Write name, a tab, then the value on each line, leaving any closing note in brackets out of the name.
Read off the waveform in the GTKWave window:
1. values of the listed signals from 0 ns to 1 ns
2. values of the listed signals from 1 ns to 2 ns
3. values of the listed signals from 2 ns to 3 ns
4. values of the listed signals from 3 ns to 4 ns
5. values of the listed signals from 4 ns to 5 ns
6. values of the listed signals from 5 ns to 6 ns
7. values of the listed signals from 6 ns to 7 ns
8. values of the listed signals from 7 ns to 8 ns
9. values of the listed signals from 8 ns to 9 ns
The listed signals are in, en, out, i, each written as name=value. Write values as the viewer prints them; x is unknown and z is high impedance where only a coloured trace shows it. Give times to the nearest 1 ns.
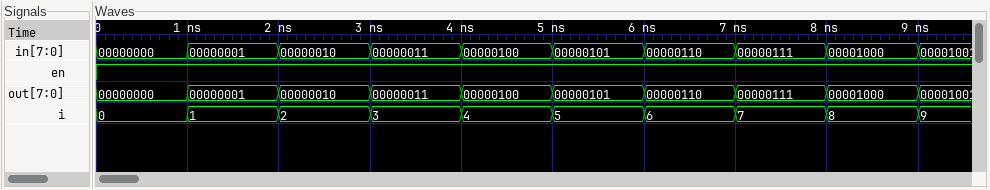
values of the listed signals from 0 ns to 1 ns	in=00000000, en=1, out=00000000, i=0
values of the listed signals from 1 ns to 2 ns	in=00000001, en=1, out=00000001, i=1
values of the listed signals from 2 ns to 3 ns	in=00000010, en=1, out=00000010, i=2
values of the listed signals from 3 ns to 4 ns	in=00000011, en=1, out=00000011, i=3
values of the listed signals from 4 ns to 5 ns	in=00000100, en=1, out=00000100, i=4
values of the listed signals from 5 ns to 6 ns	in=00000101, en=1, out=00000101, i=5
values of the listed signals from 6 ns to 7 ns	in=00000110, en=1, out=00000110, i=6
values of the listed signals from 7 ns to 8 ns	in=00000111, en=1, out=00000111, i=7
values of the listed signals from 8 ns to 9 ns	in=00001000, en=1, out=00001000, i=8
